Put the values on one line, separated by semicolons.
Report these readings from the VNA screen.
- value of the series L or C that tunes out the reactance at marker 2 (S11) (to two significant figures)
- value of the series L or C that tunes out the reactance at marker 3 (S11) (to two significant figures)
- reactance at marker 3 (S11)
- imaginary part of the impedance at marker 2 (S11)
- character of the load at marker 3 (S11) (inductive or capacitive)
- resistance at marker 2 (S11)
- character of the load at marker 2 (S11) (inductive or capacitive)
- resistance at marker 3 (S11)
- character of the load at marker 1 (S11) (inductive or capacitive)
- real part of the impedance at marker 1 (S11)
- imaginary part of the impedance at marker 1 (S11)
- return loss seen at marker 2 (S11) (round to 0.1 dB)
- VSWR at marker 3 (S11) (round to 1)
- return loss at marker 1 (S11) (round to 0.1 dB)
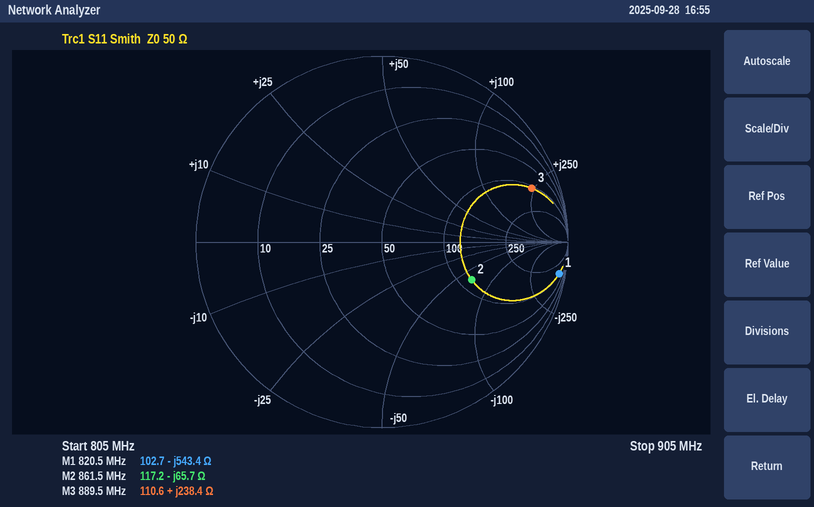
12 nH; 750 fF; +238.4 Ω; -65.7 Ω; inductive; 117.2 Ω; capacitive; 110.6 Ω; capacitive; 102.7 Ω; -543.4 Ω; 5.6 dB; 13; 0.3 dB
